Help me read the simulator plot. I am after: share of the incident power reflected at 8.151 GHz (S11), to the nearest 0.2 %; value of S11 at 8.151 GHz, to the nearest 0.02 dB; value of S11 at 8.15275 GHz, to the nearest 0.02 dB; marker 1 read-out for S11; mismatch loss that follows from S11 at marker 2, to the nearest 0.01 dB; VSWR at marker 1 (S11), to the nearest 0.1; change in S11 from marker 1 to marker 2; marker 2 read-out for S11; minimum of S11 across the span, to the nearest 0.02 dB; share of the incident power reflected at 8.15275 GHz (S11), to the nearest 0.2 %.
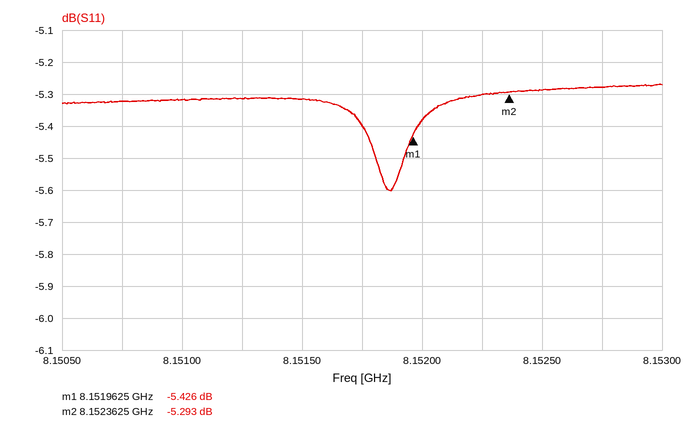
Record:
29.4 %
-5.32 dB
-5.28 dB
-5.426 dB
1.52 dB
3.3
0.133 dB
-5.293 dB
-5.60 dB
29.6 %
